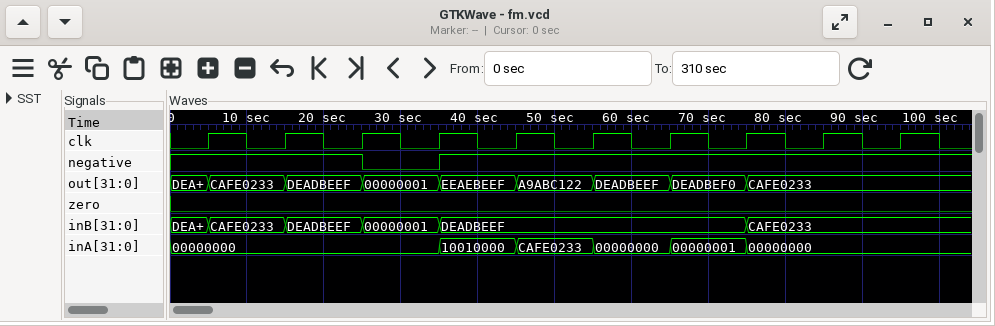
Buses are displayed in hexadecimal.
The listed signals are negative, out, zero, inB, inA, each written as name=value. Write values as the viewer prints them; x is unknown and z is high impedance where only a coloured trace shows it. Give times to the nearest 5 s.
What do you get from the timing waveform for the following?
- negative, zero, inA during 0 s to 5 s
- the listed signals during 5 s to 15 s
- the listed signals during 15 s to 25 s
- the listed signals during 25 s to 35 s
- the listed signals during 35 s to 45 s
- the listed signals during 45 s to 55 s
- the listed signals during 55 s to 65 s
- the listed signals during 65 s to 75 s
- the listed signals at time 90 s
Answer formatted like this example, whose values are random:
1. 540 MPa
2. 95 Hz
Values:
1. negative=1, zero=0, inA=00000000
2. negative=1, out=CAFE0233, zero=0, inB=CAFE0233, inA=00000000
3. negative=1, out=DEADBEEF, zero=0, inB=DEADBEEF, inA=00000000
4. negative=0, out=00000001, zero=0, inB=00000001, inA=00000000
5. negative=1, out=EEAEBEEF, zero=0, inB=DEADBEEF, inA=10010000
6. negative=1, out=A9ABC122, zero=0, inB=DEADBEEF, inA=CAFE0233
7. negative=1, out=DEADBEEF, zero=0, inB=DEADBEEF, inA=00000000
8. negative=1, out=DEADBEF0, zero=0, inB=DEADBEEF, inA=00000001
9. negative=1, out=CAFE0233, zero=0, inB=CAFE0233, inA=00000000
